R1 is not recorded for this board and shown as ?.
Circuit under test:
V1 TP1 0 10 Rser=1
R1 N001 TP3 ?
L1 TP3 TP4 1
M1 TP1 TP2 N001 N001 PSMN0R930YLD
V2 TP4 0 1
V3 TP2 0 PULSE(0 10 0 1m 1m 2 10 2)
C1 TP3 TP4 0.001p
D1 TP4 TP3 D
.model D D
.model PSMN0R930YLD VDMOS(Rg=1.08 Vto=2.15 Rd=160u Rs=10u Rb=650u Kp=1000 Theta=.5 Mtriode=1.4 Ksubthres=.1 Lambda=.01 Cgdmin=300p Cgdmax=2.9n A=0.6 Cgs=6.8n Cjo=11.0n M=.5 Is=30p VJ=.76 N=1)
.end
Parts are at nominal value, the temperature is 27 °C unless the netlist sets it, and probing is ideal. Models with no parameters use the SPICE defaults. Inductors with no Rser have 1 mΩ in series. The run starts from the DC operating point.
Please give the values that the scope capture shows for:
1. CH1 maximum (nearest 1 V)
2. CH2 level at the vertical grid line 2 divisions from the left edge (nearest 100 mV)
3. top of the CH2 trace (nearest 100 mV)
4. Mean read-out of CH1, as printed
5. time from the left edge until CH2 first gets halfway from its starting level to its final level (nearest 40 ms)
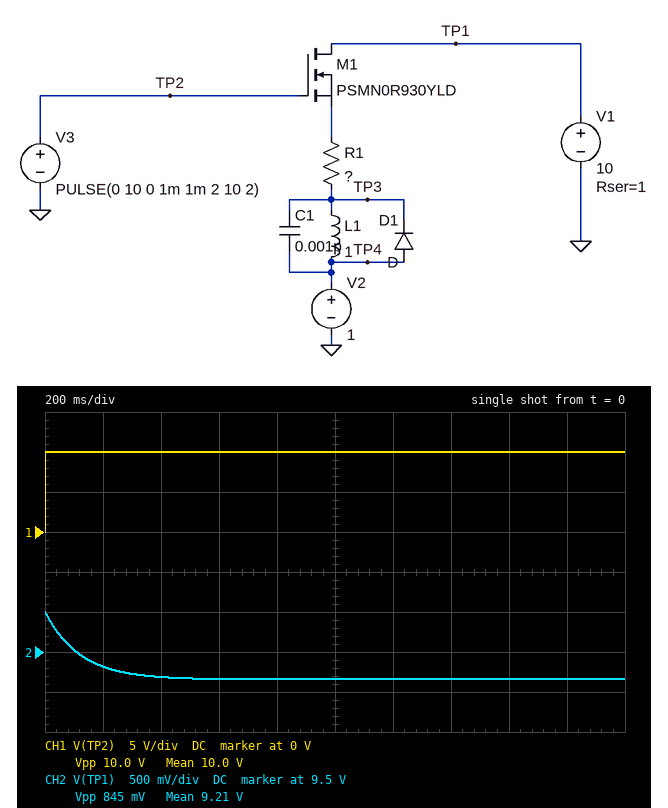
10 V
9.2 V
10.0 V
10.0 V
80 ms
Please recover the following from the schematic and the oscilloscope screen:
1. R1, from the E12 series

8.2 Ω
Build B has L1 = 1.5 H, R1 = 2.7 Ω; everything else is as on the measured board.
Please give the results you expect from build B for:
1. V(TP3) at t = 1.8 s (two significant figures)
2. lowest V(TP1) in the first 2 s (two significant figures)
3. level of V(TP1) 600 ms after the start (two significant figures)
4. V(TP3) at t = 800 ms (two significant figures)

1.2 V
7.6 V
8.3 V
2.6 V
